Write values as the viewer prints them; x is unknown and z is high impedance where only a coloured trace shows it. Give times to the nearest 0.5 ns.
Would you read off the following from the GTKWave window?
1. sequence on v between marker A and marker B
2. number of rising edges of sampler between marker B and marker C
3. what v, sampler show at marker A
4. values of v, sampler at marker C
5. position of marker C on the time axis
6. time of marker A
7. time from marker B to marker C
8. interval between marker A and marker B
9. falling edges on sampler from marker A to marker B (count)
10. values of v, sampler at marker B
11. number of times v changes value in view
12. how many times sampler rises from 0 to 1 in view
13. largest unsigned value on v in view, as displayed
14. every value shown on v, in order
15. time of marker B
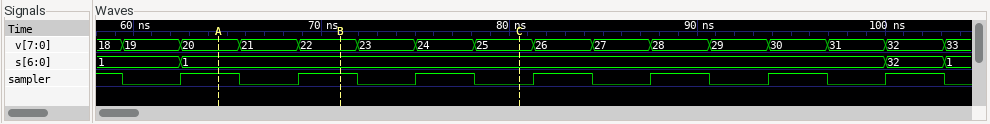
20, 21, 22
1
v=20, sampler=1
v=25, sampler=0
80.5 ns
64.5 ns
9.5 ns
6.5 ns
1
v=22, sampler=1
15
7
33
18, 19, 20, 21, 22, 23, 24, 25, 26, 27, 28, 29, 30, 31, 32, 33
71 ns
